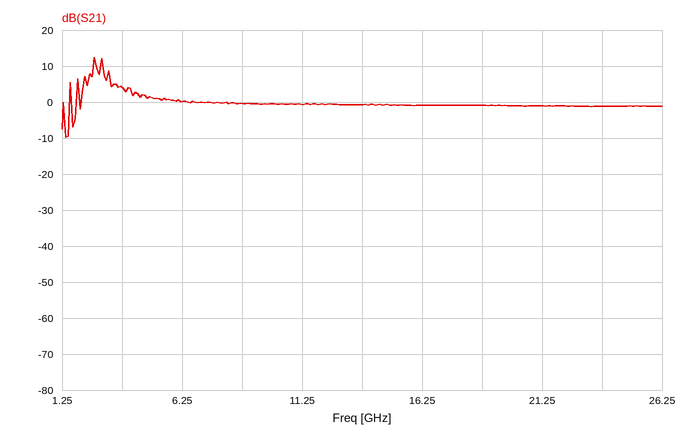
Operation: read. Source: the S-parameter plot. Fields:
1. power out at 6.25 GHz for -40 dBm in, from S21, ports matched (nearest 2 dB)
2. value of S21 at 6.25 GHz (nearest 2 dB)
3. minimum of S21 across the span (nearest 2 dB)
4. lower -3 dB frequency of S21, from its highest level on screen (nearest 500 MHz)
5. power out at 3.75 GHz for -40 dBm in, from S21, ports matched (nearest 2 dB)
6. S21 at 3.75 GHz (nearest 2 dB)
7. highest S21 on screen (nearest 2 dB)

-40 dBm
0 dB
-10 dB
2.5 GHz
-36 dBm
4 dB
12 dB
